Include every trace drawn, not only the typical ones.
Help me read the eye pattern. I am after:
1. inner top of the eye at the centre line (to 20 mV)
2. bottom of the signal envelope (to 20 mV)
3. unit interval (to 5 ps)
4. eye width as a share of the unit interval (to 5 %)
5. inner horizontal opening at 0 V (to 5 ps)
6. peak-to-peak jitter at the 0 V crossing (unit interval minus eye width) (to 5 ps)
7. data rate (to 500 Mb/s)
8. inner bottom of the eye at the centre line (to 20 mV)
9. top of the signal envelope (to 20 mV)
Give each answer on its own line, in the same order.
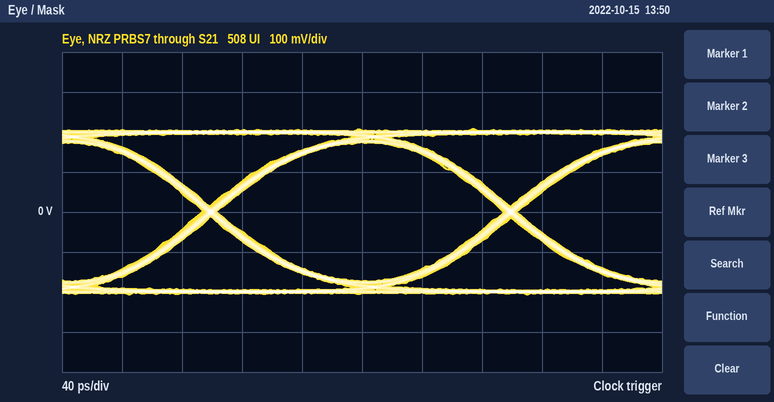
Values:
180 mV
-200 mV
200 ps
95 %
190 ps
10 ps
5.0 Gb/s
-180 mV
200 mV
